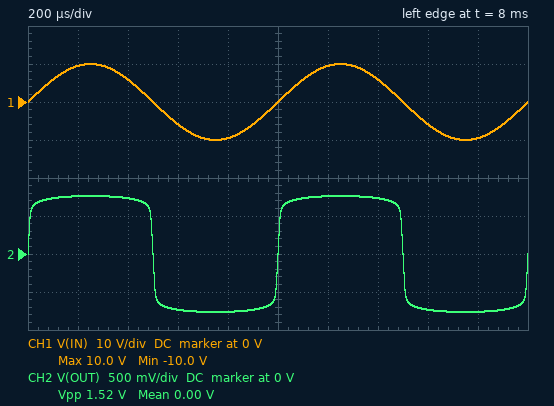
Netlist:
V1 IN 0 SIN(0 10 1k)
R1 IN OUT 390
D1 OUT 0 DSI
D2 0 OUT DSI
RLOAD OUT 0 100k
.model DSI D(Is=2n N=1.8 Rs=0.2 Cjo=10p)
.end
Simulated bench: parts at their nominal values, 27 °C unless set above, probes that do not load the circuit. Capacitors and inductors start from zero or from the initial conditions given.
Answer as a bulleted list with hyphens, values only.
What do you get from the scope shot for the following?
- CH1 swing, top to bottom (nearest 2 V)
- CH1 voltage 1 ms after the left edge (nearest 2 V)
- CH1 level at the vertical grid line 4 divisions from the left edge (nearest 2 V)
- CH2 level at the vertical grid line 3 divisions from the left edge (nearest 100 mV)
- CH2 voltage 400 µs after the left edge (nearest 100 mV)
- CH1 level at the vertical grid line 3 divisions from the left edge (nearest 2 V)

- 20 V
- 0 V
- -10 V
- -700 mV
- 700 mV
- -6 V
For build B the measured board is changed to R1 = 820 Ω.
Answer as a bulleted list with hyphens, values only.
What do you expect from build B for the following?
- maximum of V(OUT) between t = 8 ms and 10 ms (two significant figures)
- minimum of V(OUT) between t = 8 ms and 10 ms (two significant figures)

- 730 mV
- -730 mV
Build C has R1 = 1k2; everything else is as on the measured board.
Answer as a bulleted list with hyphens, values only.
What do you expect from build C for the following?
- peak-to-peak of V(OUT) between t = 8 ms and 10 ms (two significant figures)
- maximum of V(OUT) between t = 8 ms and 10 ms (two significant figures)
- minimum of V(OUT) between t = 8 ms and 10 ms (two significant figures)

- 1.4 V
- 710 mV
- -710 mV
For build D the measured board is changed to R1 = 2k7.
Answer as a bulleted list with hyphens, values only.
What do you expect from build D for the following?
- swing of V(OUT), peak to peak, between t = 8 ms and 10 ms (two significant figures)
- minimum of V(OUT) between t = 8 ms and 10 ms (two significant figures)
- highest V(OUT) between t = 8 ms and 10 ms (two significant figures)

- 1.3 V
- -670 mV
- 670 mV
